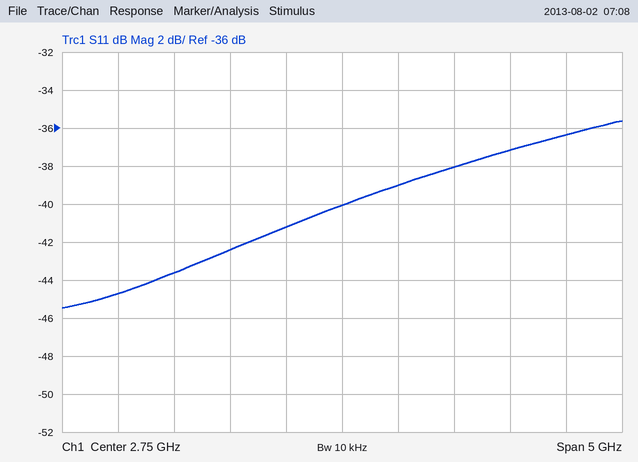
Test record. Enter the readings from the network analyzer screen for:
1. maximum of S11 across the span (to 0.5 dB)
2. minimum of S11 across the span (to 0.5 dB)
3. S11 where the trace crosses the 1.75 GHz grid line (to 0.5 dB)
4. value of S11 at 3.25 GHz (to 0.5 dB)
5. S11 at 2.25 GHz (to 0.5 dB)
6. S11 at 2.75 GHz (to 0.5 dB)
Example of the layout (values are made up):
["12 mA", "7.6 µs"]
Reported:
["-35.5 dB", "-45.5 dB", "-42.5 dB", "-39.0 dB", "-41.0 dB", "-40.0 dB"]
